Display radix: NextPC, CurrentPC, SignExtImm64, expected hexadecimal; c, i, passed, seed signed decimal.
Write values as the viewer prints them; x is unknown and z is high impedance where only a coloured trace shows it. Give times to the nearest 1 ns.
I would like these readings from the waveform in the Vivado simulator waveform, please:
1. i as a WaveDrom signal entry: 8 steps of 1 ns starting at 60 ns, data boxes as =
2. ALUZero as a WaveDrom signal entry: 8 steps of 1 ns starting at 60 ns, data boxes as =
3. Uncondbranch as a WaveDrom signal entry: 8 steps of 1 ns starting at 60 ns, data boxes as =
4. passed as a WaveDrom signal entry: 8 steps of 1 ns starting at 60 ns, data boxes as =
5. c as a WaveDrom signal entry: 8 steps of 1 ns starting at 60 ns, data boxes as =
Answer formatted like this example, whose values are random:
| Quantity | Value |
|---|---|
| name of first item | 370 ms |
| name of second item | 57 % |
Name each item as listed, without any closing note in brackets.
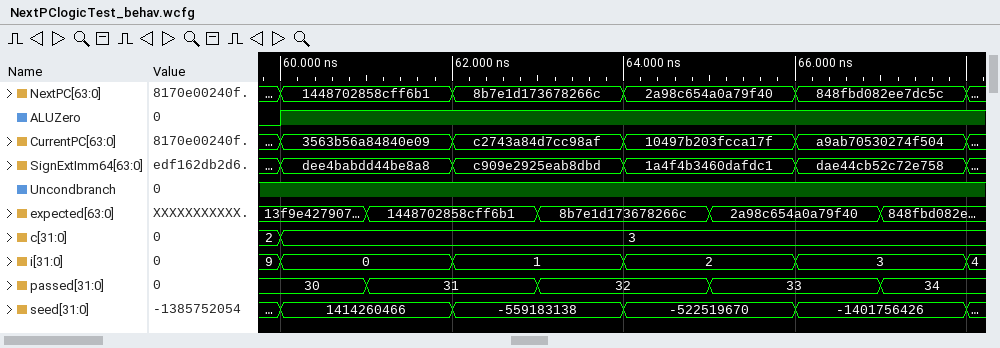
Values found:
| Quantity | Value |
|---|---|
| i as a WaveDrom signal entry: 8 steps of 1 ns starting at 60 ns, data boxes as = | {name: 'i', wave: '=.=.=.=.', data: '0 1 2 3'} |
| ALUZero as a WaveDrom signal entry: 8 steps of 1 ns starting at 60 ns, data boxes as = | {name: 'ALUZero', wave: '1.......'} |
| Uncondbranch as a WaveDrom signal entry: 8 steps of 1 ns starting at 60 ns, data boxes as = | {name: 'Uncondbranch', wave: '1.......'} |
| passed as a WaveDrom signal entry: 8 steps of 1 ns starting at 60 ns, data boxes as = | {name: 'passed', wave: '==.=.=.=', data: '30 31 32 33 34'} |
| c as a WaveDrom signal entry: 8 steps of 1 ns starting at 60 ns, data boxes as = | {name: 'c', wave: '=.......', data: '3'} |
